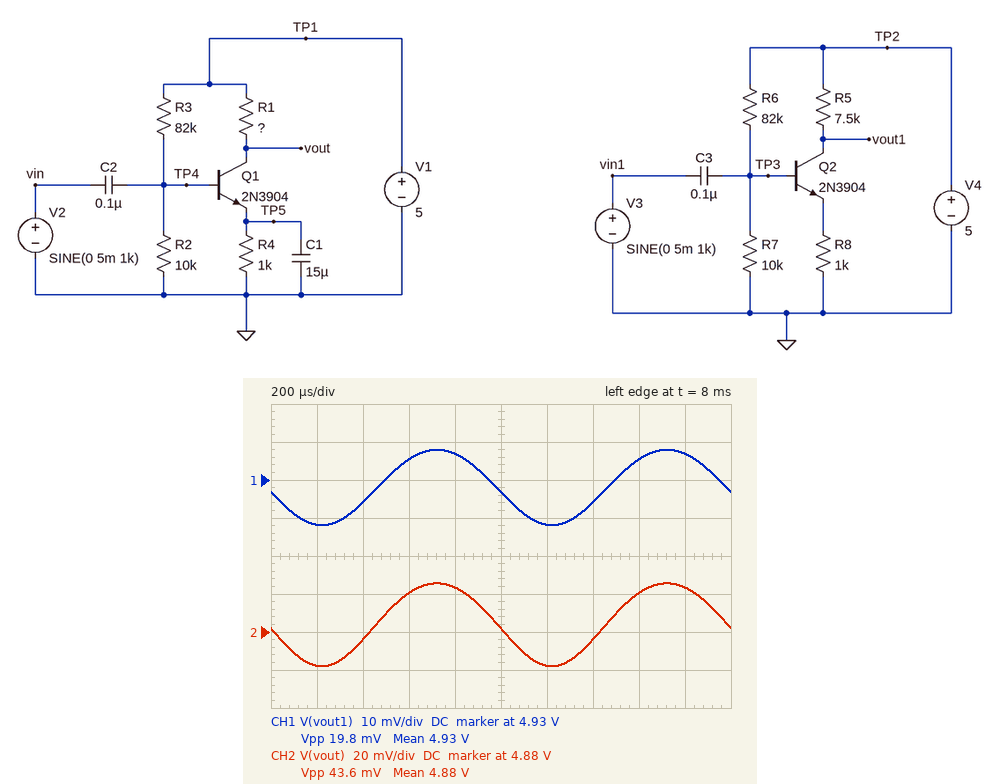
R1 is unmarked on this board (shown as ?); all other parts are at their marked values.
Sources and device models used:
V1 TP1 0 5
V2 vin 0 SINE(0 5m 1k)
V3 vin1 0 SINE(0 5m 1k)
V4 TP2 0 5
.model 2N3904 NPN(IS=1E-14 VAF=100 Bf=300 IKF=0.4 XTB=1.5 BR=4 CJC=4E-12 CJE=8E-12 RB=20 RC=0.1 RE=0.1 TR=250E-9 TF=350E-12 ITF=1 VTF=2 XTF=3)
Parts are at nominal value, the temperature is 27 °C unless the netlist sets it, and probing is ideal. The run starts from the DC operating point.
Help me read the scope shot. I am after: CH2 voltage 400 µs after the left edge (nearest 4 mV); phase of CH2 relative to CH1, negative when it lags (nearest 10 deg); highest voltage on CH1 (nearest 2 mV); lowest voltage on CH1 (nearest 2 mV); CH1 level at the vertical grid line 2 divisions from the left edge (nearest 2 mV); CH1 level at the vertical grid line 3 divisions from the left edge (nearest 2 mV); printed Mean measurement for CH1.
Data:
4.876 V
0 deg
4.938 V
4.918 V
4.924 V
4.936 V
4.93 V
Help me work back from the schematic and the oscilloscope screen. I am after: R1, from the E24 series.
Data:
12 kΩ
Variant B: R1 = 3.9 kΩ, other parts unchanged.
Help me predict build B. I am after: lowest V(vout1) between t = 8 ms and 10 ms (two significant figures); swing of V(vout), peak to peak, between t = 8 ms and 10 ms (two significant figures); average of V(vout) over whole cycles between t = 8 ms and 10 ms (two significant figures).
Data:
4.9 V
14 mV
5.0 V
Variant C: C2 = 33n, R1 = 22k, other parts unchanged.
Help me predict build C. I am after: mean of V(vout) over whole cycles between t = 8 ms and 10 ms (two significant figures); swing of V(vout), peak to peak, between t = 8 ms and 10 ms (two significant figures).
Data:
4.8 V
71 mV
